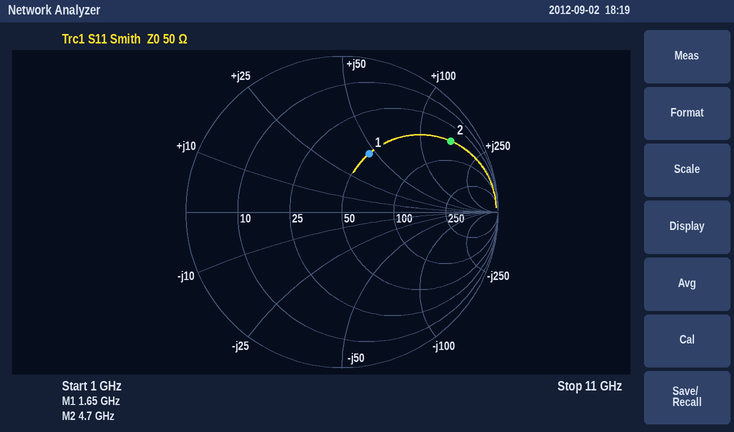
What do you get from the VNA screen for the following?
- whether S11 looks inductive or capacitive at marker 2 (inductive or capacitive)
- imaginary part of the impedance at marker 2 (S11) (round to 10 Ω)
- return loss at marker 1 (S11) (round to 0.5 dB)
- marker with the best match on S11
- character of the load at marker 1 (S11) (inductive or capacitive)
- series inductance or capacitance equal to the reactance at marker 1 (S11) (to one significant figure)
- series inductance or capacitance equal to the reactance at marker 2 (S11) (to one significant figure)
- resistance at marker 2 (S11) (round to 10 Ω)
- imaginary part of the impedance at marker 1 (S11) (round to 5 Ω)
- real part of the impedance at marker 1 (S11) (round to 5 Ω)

inductive
+150 Ω
7.5 dB
marker 1
inductive
4 nH
5 nH
50 Ω
+45 Ω
50 Ω
